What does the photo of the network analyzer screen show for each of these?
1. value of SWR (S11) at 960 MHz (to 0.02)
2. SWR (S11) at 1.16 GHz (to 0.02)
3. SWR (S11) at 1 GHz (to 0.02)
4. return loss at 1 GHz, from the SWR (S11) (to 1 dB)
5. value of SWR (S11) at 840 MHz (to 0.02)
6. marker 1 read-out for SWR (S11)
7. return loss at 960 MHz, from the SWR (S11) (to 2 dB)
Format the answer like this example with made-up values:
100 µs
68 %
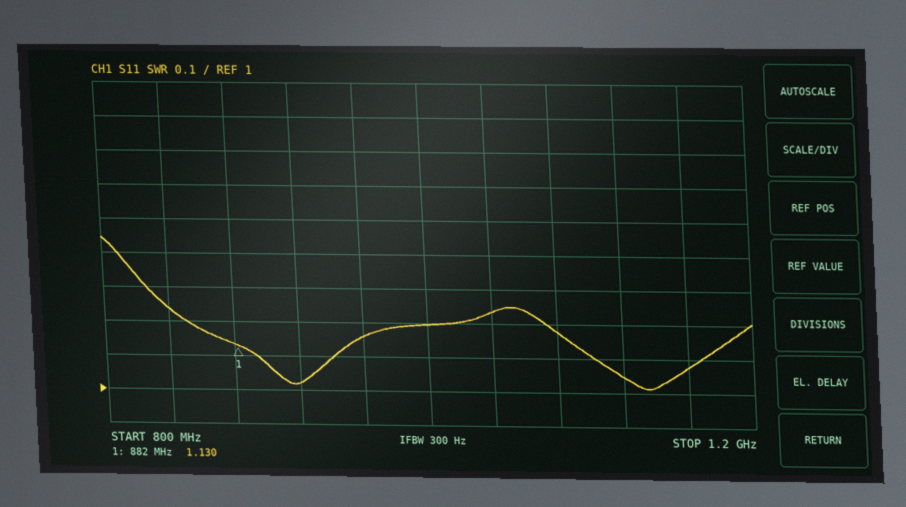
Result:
1.16
1.08
1.20
21 dB
1.24
1.130
22 dB
